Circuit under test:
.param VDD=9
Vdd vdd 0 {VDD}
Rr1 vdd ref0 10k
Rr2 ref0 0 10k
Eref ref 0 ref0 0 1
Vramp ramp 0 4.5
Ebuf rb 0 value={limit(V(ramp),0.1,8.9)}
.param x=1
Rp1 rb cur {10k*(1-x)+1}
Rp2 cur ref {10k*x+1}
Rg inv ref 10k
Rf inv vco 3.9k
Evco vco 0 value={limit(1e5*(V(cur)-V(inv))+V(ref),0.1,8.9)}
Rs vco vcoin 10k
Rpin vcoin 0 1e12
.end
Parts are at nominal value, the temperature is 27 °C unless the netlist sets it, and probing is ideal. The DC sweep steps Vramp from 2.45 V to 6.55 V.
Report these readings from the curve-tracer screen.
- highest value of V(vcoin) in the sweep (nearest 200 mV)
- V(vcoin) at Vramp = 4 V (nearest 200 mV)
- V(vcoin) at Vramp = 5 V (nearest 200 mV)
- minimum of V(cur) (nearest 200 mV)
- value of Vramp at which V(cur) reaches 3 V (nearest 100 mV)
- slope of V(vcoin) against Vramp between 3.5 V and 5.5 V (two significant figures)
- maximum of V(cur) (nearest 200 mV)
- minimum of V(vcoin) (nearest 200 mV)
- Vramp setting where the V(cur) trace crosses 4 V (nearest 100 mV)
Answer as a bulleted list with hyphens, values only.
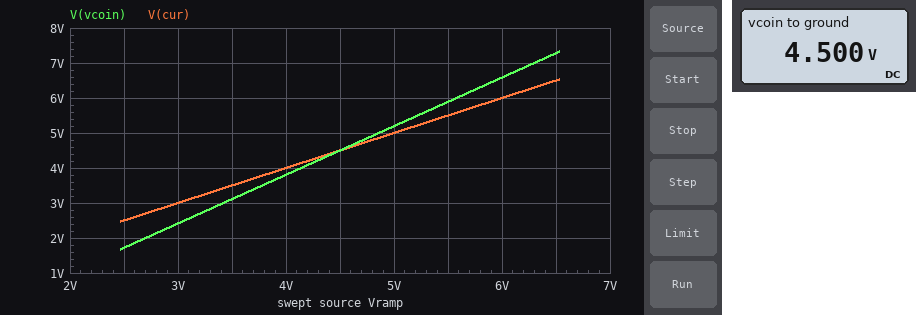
- 7.4 V
- 3.8 V
- 5.2 V
- 2.4 V
- 3.0 V
- 1.4 V/V
- 6.6 V
- 1.6 V
- 4.0 V
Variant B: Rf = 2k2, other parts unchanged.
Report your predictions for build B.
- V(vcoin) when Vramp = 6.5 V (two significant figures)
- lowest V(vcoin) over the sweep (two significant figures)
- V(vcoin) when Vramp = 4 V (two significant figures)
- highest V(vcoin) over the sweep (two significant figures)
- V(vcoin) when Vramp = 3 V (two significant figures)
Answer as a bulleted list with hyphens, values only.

- 6.9 V
- 2.0 V
- 3.9 V
- 7.0 V
- 2.7 V
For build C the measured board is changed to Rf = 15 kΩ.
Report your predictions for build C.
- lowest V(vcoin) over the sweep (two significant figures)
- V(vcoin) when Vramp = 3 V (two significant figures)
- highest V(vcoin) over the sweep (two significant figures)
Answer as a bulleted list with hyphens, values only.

- 100 mV
- 750 mV
- 8.9 V
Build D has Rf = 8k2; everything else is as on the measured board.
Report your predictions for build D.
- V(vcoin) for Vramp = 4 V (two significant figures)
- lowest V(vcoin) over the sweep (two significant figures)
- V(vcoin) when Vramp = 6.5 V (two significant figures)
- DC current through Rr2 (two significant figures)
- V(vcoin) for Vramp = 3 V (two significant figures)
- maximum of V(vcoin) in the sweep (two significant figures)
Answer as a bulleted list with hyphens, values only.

- 3.6 V
- 780 mV
- 8.1 V
- 450 µA
- 1.8 V
- 8.2 V
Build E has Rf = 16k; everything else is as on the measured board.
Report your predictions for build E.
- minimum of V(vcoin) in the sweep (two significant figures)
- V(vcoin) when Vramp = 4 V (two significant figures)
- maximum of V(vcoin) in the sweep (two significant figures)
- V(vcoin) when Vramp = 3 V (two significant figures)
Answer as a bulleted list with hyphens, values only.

- 100 mV
- 3.2 V
- 8.9 V
- 600 mV
